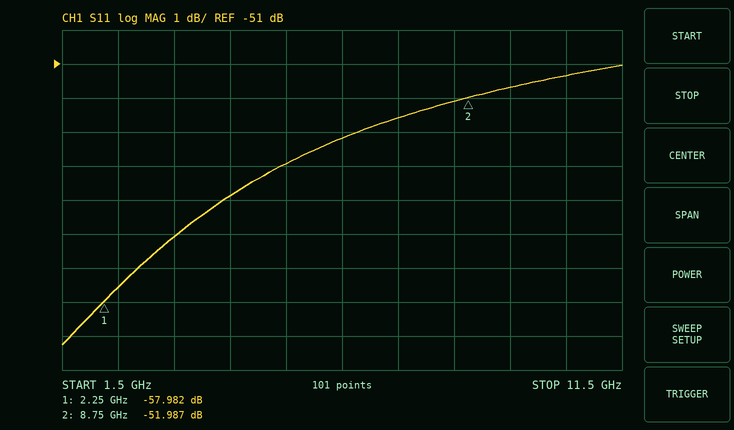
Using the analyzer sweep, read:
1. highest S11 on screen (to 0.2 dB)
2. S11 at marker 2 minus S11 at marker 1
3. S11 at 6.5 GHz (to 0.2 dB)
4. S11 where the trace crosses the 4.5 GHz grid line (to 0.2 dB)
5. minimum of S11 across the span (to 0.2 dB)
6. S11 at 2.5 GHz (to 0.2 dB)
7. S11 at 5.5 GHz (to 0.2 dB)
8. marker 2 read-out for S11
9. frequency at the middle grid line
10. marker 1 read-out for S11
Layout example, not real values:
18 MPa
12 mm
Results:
-51.0 dB
5.995 dB
-53.2 dB
-54.8 dB
-59.2 dB
-57.6 dB
-54.0 dB
-51.987 dB
6.5 GHz
-57.982 dB
